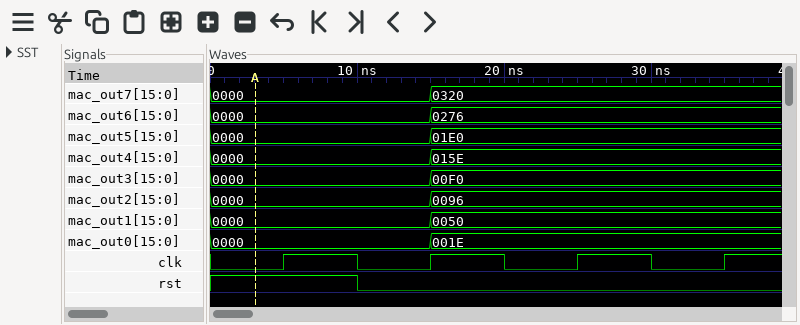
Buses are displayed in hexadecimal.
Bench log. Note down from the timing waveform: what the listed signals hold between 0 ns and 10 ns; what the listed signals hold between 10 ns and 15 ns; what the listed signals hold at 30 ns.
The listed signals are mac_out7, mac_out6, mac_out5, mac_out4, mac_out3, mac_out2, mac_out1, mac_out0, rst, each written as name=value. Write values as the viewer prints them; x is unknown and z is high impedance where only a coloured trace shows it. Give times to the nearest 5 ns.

mac_out7=0000, mac_out6=0000, mac_out5=0000, mac_out4=0000, mac_out3=0000, mac_out2=0000, mac_out1=0000, mac_out0=0000, rst=1
mac_out7=0000, mac_out6=0000, mac_out5=0000, mac_out4=0000, mac_out3=0000, mac_out2=0000, mac_out1=0000, mac_out0=0000, rst=0
mac_out7=0320, mac_out6=0276, mac_out5=01E0, mac_out4=015E, mac_out3=00F0, mac_out2=0096, mac_out1=0050, mac_out0=001E, rst=0
